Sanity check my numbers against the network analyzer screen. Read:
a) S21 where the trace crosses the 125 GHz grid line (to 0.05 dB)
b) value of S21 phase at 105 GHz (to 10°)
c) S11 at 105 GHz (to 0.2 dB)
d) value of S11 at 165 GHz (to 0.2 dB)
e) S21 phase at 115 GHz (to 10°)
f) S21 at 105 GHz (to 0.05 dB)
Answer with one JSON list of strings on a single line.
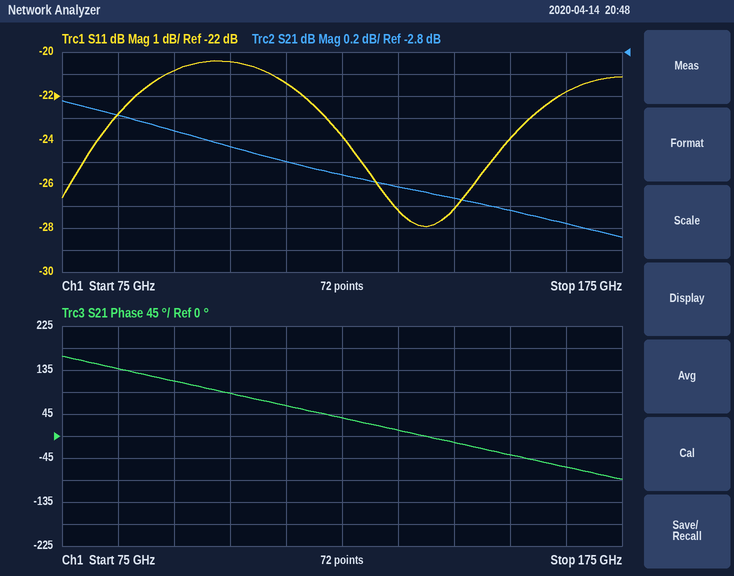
["-3.90 dB", "90°", "-20.4 dB", "-21.8 dB", "60°", "-3.65 dB"]
